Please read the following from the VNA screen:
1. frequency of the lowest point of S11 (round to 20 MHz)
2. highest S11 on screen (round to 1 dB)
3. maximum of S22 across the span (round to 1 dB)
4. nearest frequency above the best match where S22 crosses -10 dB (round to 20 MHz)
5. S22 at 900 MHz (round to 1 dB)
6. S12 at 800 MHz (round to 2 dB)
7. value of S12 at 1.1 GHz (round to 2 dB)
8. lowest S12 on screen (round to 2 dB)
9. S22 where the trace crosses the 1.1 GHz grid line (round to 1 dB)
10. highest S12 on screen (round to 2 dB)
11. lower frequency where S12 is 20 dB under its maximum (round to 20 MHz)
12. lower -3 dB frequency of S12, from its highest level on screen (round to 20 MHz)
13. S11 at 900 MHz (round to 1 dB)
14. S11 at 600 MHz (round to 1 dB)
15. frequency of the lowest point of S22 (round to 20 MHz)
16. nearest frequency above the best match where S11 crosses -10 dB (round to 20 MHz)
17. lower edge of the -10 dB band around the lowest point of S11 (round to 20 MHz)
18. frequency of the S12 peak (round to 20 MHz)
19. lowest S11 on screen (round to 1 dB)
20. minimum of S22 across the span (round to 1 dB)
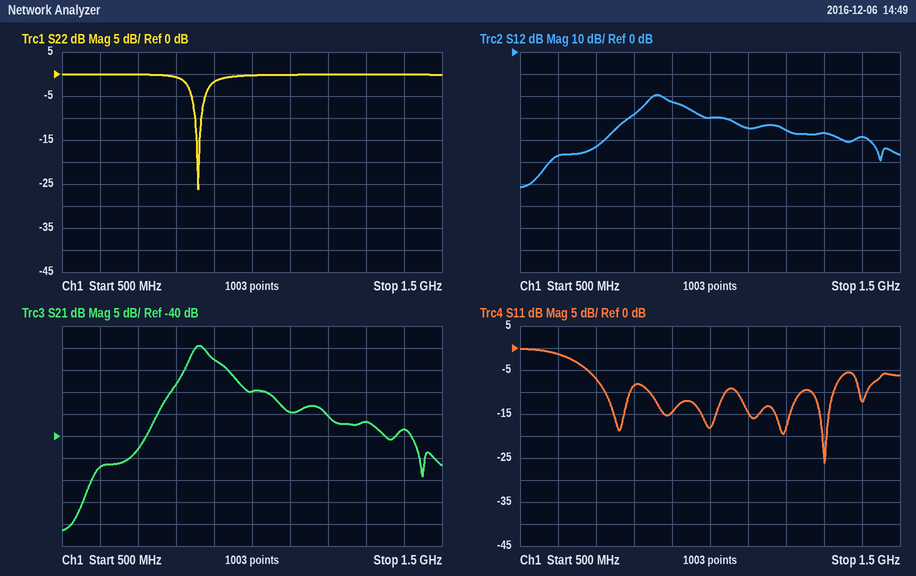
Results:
1.30 GHz
0 dB
0 dB
860 MHz
-2 dB
-28 dB
-34 dB
-62 dB
0 dB
-20 dB
720 MHz
840 MHz
-15 dB
-1 dB
860 MHz
1.32 GHz
1.26 GHz
860 MHz
-26 dB
-26 dB
